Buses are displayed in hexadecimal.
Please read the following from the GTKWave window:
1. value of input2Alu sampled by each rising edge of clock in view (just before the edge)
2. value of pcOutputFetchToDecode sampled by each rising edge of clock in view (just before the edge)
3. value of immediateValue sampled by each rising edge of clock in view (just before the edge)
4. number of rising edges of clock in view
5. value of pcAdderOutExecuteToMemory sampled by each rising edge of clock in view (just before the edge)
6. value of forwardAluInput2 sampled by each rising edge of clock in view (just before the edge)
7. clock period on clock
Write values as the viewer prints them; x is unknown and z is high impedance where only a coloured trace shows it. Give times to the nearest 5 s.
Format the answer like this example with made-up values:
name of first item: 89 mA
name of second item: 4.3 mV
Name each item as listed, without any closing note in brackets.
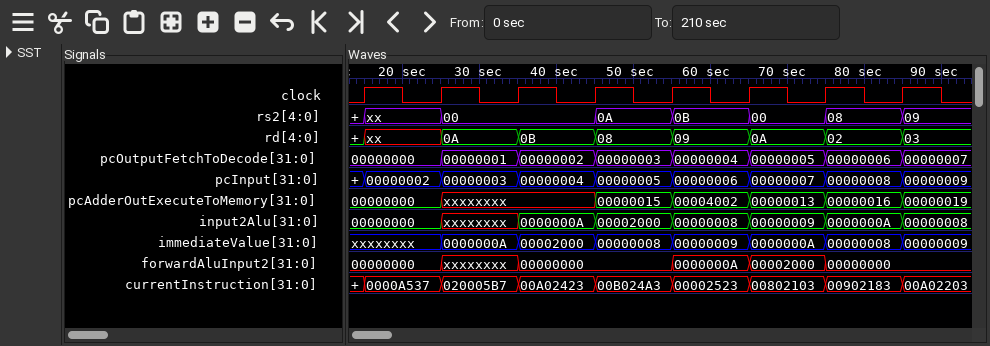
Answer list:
value of input2Alu sampled by each rising edge of clock in view: 00000000, 00000000, xxxxxxxx, 0000000A, 00002000, 00000008, 00000009, 0000000A
value of pcOutputFetchToDecode sampled by each rising edge of clock in view: 00000000, 00000000, 00000001, 00000002, 00000003, 00000004, 00000005, 00000006
value of immediateValue sampled by each rising edge of clock in view: xxxxxxxx, xxxxxxxx, 0000000A, 00002000, 00000008, 00000009, 0000000A, 00000008
number of rising edges of clock in view: 8
value of pcAdderOutExecuteToMemory sampled by each rising edge of clock in view: 00000000, 00000000, xxxxxxxx, xxxxxxxx, 00000015, 00004002, 00000013, 00000016
value of forwardAluInput2 sampled by each rising edge of clock in view: 00000000, 00000000, xxxxxxxx, 00000000, 00000000, 0000000A, 00002000, 00000000
clock period on clock: 10 s
